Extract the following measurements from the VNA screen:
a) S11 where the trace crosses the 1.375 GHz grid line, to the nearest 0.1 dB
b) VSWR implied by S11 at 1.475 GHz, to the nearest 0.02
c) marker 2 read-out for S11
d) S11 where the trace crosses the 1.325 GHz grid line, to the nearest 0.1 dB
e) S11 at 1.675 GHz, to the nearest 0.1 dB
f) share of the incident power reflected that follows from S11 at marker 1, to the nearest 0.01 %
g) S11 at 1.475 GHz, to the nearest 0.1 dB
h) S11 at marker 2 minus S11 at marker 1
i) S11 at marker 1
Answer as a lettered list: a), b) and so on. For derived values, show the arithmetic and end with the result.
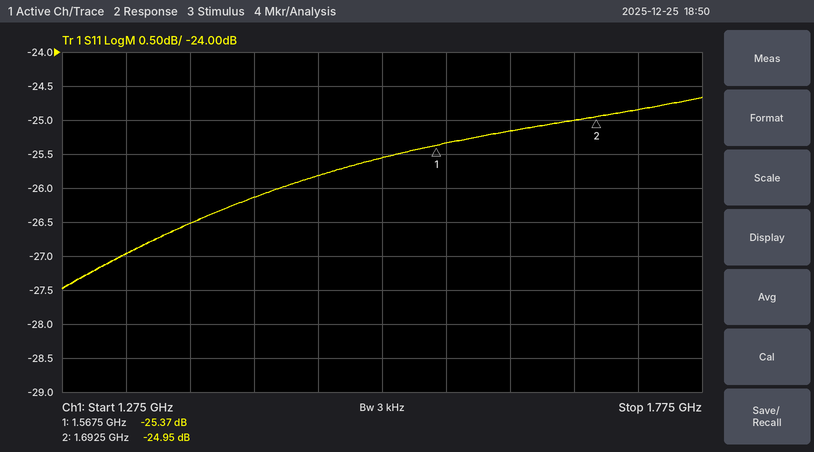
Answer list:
a) -26.5 dB
b) |Γ| = 10^(-25.8/20) = 0.0513; VSWR = (1 + 0.0513)/(1 − 0.0513) ≈ 1.11, so 1.10 to the nearest 0.02
c) -24.95 dB
d) -27.0 dB
e) -25.0 dB
f) 10^(-25.37/10) ≈ 0.29 %
g) -25.8 dB
h) -24.95 − (-25.37) = 0.42 dB
i) -25.37 dB
